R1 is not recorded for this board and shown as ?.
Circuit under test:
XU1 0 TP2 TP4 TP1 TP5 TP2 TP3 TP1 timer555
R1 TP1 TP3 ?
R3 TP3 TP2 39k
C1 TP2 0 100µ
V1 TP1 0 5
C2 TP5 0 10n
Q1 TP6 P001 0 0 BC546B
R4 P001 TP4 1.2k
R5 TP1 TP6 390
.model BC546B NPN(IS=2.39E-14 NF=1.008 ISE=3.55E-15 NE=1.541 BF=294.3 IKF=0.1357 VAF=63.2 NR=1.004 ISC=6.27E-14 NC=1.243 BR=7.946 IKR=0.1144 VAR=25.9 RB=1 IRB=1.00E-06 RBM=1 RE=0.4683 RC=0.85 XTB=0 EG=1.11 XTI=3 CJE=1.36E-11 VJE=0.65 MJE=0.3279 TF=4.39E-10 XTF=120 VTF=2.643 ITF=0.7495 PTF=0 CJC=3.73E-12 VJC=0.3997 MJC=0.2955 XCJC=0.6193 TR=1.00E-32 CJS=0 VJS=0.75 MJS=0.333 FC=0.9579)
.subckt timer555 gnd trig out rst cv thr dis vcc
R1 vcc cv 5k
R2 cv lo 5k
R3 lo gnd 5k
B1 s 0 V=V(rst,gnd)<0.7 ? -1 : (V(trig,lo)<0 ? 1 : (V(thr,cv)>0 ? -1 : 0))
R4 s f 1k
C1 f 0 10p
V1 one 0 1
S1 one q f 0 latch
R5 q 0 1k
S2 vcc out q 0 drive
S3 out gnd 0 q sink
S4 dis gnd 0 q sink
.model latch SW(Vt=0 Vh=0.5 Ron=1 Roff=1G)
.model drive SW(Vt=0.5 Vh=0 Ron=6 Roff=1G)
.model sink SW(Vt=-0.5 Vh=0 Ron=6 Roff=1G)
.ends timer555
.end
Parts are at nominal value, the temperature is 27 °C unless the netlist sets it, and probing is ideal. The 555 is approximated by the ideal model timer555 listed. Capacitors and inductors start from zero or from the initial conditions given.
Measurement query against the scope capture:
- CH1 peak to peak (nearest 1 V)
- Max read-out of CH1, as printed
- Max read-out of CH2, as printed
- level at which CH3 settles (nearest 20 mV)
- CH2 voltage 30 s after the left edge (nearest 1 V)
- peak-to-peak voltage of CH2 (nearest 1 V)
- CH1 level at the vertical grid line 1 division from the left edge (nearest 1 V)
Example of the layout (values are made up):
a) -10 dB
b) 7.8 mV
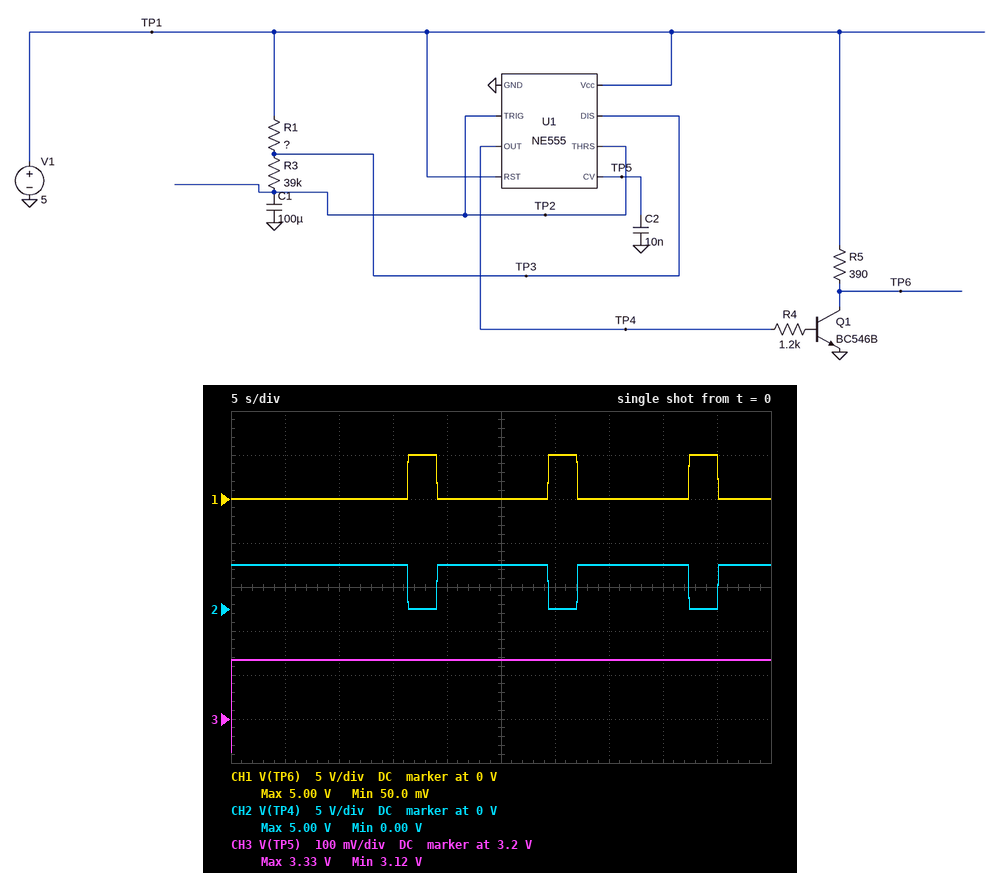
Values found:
a) 5 V
b) 5.00 V
c) 5.00 V
d) 3.34 V
e) 0 V
f) 5 V
g) 0 V
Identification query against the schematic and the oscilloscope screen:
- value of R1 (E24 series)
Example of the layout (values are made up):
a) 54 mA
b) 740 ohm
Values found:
a) 110 kΩ
